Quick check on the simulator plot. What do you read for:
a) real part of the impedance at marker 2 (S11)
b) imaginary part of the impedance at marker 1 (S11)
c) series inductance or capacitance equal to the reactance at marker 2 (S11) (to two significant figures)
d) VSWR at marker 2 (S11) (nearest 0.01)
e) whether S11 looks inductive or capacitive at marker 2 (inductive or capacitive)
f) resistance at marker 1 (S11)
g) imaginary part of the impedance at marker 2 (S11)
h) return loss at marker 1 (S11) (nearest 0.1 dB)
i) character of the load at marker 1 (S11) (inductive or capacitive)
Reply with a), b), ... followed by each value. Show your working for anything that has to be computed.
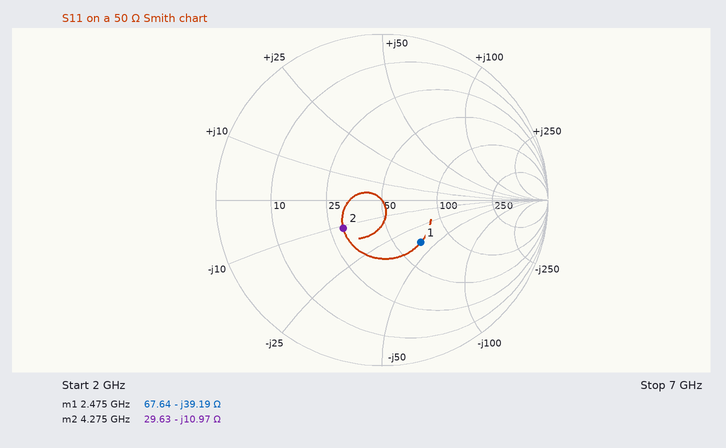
a) 29.63 Ω
b) -39.19 Ω
c) C = 1/(2π × 4.275 GHz × 10.97 Ω) ≈ 3.4 pF
d) 1.81
e) capacitive
f) 67.64 Ω
g) -10.97 Ω
h) 9.2 dB
i) capacitive
